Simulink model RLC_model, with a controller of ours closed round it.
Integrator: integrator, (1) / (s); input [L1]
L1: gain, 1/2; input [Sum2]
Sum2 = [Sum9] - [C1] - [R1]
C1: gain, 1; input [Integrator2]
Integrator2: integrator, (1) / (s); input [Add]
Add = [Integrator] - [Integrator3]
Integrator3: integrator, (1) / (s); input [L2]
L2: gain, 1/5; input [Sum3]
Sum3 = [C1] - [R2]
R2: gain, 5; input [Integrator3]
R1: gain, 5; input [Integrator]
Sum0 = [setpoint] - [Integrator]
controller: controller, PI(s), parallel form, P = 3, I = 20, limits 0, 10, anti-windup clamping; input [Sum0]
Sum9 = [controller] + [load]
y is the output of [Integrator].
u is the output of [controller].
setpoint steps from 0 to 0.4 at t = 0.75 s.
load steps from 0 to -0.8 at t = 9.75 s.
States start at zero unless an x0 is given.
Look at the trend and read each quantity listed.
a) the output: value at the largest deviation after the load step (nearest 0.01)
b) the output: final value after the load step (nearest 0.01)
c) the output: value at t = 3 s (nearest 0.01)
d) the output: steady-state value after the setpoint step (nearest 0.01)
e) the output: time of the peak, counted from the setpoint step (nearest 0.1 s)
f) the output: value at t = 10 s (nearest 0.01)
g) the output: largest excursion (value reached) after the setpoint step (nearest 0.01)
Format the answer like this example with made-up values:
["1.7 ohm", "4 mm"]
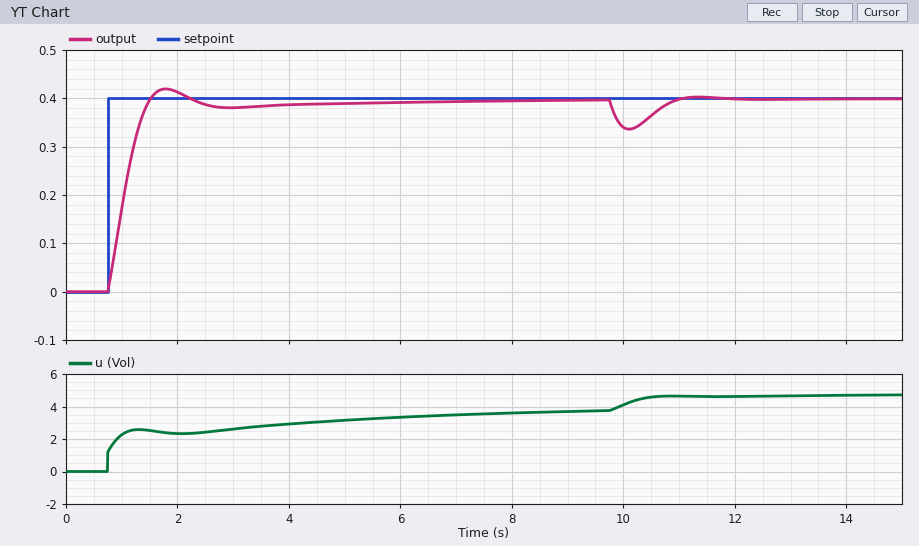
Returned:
["0.34", "0.40", "0.38", "0.40", "1.0 s", "0.34", "0.42"]
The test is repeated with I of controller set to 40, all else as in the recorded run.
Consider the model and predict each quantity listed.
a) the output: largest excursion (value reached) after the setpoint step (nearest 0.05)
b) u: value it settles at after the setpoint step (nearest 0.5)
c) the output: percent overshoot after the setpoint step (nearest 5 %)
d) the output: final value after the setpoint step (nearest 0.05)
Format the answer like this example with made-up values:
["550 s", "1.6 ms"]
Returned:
["0.50", "4.0", "20 %", "0.40"]
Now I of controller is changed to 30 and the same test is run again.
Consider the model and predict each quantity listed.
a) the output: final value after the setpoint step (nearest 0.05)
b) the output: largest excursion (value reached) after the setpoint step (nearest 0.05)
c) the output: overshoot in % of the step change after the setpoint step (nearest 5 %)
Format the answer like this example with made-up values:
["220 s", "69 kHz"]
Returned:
["0.40", "0.45", "15 %"]
